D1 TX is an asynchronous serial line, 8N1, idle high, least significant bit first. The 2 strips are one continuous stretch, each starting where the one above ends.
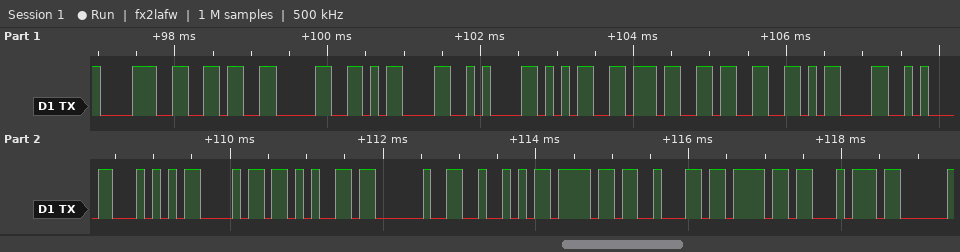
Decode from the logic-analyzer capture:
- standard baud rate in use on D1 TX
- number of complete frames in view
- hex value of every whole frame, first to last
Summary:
9600 baud
19
38 36 30 0D 0A 35 37 33 0D 0A 54 68 65 20 52 6F 62 6F 74
